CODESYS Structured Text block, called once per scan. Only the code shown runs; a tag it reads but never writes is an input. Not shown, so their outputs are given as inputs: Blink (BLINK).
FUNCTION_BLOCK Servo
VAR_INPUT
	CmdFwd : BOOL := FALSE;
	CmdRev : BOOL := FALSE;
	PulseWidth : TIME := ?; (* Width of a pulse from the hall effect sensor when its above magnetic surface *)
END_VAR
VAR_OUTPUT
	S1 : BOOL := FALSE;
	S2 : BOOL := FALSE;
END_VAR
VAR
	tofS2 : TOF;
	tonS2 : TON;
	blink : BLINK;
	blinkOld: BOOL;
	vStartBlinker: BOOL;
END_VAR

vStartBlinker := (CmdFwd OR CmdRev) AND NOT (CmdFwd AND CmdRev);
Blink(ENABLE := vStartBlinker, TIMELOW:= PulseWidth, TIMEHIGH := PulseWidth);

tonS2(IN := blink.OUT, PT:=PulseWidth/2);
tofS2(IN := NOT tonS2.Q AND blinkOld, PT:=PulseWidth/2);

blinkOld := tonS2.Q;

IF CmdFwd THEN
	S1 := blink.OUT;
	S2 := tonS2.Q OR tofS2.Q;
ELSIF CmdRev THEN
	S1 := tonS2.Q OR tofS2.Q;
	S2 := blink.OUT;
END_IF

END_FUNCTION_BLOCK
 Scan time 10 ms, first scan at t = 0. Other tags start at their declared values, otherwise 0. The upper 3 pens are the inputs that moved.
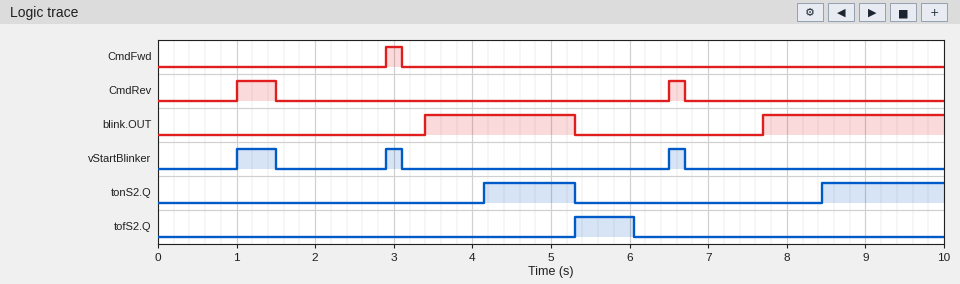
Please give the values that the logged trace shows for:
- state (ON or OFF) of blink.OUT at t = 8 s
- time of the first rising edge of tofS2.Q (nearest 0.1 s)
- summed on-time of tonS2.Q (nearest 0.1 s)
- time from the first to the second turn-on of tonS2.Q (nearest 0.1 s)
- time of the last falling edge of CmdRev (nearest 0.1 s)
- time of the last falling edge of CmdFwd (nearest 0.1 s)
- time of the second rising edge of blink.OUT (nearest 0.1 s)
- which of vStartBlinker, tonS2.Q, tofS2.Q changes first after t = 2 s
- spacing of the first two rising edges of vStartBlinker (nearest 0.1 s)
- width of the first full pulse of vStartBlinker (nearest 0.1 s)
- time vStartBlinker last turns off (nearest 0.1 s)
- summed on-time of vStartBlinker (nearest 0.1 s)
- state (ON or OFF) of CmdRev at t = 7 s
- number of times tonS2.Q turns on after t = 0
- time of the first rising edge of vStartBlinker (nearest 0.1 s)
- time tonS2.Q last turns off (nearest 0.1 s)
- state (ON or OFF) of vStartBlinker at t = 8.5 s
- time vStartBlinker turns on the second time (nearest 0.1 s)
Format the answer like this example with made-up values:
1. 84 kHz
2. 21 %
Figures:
1. ON
2. 5.3 s
3. 2.7 s
4. 4.3 s
5. 6.7 s
6. 3.1 s
7. 7.7 s
8. vStartBlinker
9. 1.9 s
10. 0.5 s
11. 6.7 s
12. 0.9 s
13. OFF
14. 2
15. 1.0 s
16. 5.3 s
17. OFF
18. 2.9 s
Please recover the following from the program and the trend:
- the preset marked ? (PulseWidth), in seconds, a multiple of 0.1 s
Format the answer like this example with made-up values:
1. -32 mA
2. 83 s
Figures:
1. 1.5 s
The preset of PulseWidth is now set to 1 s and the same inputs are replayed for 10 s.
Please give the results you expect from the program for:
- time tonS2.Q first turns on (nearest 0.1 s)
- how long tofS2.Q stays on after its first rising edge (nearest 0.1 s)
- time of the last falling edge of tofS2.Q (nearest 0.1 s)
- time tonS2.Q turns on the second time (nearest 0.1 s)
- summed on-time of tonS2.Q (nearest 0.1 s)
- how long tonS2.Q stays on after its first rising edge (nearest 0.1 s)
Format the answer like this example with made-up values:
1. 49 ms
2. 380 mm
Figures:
1. 3.9 s
2. 0.5 s
3. 5.8 s
4. 8.2 s
5. 3.2 s
6. 1.4 s
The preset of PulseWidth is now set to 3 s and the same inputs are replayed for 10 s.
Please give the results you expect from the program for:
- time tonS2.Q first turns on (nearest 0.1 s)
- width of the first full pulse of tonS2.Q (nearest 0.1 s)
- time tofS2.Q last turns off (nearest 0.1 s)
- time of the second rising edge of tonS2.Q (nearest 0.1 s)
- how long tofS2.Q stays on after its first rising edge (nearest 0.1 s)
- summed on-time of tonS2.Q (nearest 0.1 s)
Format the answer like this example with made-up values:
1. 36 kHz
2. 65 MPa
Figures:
1. 4.9 s
2. 0.4 s
3. 6.8 s
4. 9.2 s
5. 1.5 s
6. 1.2 s
